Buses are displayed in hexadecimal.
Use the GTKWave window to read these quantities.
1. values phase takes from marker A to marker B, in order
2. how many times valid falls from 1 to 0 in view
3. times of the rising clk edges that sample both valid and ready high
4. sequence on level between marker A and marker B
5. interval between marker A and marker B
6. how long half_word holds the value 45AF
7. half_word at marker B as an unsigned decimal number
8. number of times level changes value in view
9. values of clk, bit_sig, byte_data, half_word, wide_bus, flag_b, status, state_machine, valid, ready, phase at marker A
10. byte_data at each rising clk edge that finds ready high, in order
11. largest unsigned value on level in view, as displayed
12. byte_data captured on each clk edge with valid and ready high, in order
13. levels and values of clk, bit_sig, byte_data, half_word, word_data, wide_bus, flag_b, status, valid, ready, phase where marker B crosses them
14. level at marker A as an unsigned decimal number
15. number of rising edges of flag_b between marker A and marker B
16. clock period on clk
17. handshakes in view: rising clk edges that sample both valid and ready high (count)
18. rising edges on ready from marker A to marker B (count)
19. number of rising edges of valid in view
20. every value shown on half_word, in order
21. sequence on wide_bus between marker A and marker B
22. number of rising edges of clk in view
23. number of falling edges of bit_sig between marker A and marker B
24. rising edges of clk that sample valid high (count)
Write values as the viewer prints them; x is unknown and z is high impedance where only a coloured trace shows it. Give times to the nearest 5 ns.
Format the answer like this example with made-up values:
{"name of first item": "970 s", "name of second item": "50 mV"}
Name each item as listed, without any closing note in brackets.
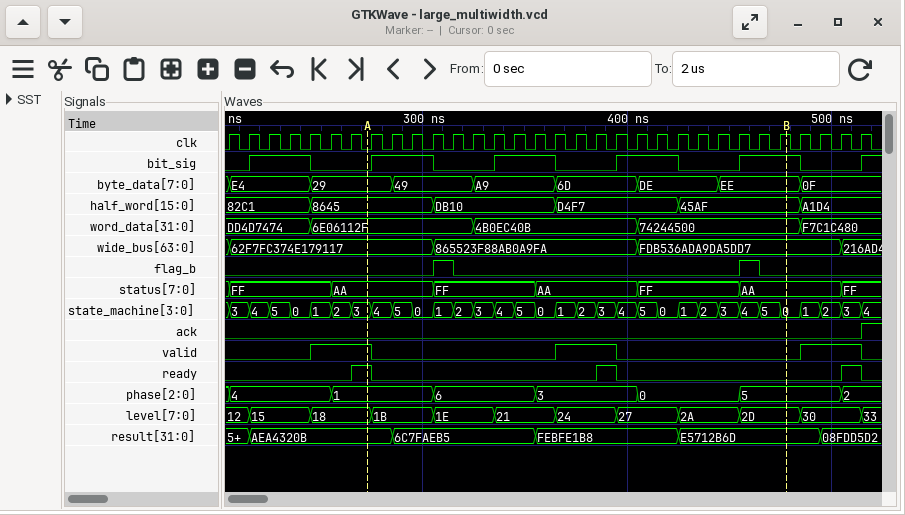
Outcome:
{"values phase takes from marker A to marker B, in order": "1, 6, 3, 0, 5", "how many times valid falls from 1 to 0 in view": "3", "times of the rising clk edges that sample both valid and ready high": "275 ns, 395 ns, 515 ns", "sequence on level between marker A and marker B": "18, 1B, 1E, 21, 24, 27, 2A, 2D", "interval between marker A and marker B": "205 ns", "how long half_word holds the value 45AF": "60 ns", "half_word at marker B as an unsigned decimal number": "17839", "number of times level changes value in view": "11", "values of clk, bit_sig, byte_data, half_word, wide_bus, flag_b, status, state_machine, valid, ready, phase at marker A": "clk=0, bit_sig=0, byte_data=29, half_word=8645, wide_bus=62F7FC374E179117, flag_b=0, status=AA, state_machine=3, valid=1, ready=1, phase=1", "byte_data at each rising clk edge that finds ready high, in order": "29, 6D, 0F", "largest unsigned value on level in view, as displayed": "33", "byte_data captured on each clk edge with valid and ready high, in order": "29, 6D, 0F", "levels and values of clk, bit_sig, byte_data, half_word, word_data, wide_bus, flag_b, status, valid, ready, phase where marker B crosses them": "clk=1, bit_sig=1, byte_data=EE, half_word=45AF, word_data=74244500, wide_bus=FDB536ADA9DA5DD7, flag_b=0, status=AA, valid=0, ready=0, phase=5", "level at marker A as an unsigned decimal number": "24", "number of rising edges of flag_b between marker A and marker B": "2", "clock period on clk": "10 ns", "handshakes in view: rising clk edges that sample both valid and ready high": "3", "rising edges on ready from marker A to marker B": "1", "number of rising edges of valid in view": "3", "every value shown on half_word, in order": "82C1, 8645, DB10, D4F7, 45AF, A1D4", "sequence on wide_bus between marker A and marker B": "62F7FC374E179117, 865523F88AB0A9FA, FDB536ADA9DA5DD7", "number of rising edges of clk in view": "32", "number of falling edges of bit_sig between marker A and marker B": "3", "rising edges of clk that sample valid high": "9"}
